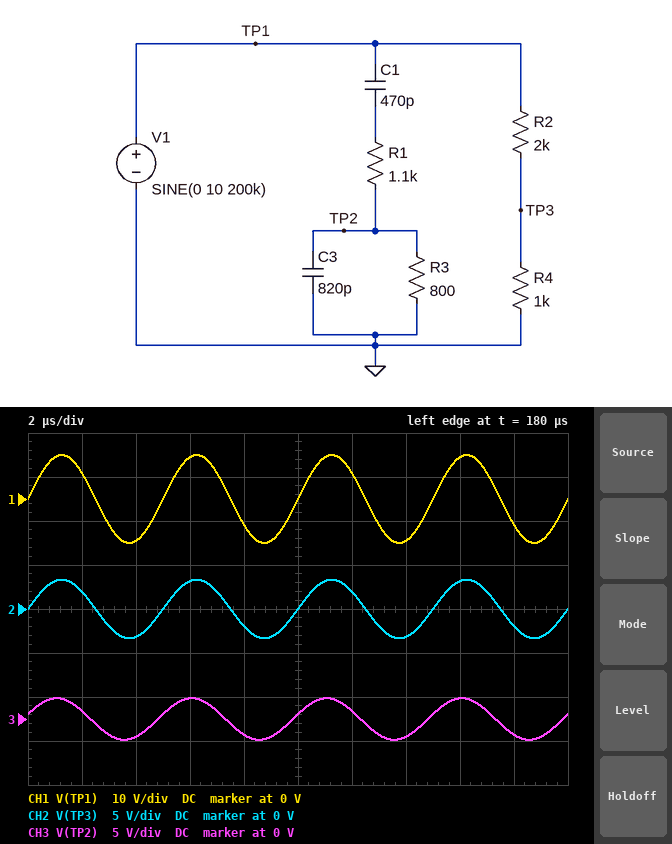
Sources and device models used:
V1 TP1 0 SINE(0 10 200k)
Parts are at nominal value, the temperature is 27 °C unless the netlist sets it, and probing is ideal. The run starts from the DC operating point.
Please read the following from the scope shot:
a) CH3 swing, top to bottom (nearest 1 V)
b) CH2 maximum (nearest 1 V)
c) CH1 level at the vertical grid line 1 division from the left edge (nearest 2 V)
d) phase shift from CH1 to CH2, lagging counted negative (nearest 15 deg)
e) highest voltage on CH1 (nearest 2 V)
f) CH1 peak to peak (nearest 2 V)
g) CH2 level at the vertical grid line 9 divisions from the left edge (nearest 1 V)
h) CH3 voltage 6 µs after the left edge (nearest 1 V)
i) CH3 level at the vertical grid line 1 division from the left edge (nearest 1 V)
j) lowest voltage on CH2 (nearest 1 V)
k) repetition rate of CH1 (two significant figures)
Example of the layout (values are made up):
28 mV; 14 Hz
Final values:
5 V; 3 V; 6 V; 0 deg; 10 V; 20 V; -2 V; 2 V; 1 V; -3 V; 200 kHz
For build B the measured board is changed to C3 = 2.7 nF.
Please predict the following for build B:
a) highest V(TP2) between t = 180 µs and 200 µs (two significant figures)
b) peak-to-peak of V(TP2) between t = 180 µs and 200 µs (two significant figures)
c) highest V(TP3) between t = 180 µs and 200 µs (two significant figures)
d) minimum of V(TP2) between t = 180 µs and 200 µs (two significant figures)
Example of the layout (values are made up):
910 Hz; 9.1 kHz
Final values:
1.2 V; 2.4 V; 3.3 V; -1.2 V
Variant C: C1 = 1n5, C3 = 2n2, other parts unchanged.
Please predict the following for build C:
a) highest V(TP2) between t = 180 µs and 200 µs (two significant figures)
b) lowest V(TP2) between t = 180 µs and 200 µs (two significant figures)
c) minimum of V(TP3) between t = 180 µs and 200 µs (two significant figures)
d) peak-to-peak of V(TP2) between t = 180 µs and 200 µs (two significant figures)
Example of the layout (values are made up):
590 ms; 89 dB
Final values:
2.2 V; -2.2 V; -3.3 V; 4.4 V
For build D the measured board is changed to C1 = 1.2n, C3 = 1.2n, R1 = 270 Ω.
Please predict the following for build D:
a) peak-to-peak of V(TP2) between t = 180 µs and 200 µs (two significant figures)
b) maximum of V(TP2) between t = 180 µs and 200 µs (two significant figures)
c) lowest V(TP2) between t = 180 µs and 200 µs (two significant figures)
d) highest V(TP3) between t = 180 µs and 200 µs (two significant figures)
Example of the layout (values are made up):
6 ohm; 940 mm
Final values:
8.4 V; 4.2 V; -4.2 V; 3.3 V
